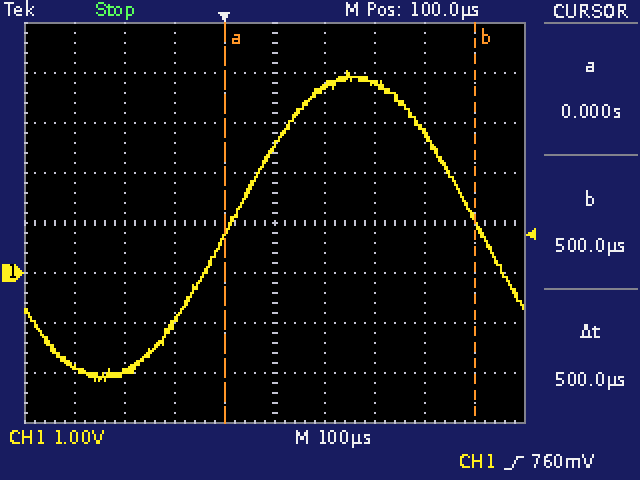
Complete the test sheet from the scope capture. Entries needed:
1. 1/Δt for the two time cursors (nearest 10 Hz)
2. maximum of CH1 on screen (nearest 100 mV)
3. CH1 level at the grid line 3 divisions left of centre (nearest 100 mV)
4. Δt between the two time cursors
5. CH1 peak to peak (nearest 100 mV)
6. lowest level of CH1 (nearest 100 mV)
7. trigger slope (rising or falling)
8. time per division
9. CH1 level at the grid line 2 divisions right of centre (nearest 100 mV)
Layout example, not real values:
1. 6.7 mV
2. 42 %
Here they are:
1. 2.00 kHz
2. 4.0 V
3. -2.0 V
4. 500 µs
5. 6.2 V
6. -2.2 V
7. rising
8. 100 µs
9. 3.8 V
